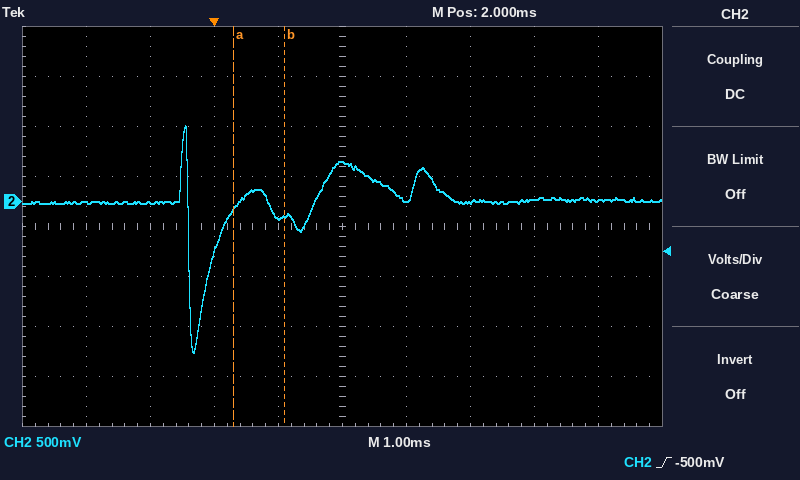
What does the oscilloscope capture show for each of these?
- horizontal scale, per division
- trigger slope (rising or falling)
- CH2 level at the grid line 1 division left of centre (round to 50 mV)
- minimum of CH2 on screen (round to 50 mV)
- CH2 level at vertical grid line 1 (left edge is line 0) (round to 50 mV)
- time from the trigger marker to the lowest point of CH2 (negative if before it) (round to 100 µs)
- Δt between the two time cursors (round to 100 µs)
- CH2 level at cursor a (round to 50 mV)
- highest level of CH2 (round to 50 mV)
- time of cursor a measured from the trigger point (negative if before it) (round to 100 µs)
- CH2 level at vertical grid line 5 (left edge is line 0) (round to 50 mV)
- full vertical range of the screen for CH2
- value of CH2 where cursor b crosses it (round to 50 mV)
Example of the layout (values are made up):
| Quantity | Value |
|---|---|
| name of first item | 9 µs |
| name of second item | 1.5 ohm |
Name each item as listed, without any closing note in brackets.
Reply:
| Quantity | Value |
|---|---|
| horizontal scale, per division | 1 ms |
| trigger slope | rising |
| CH2 level at the grid line 1 division left of centre | -150 mV |
| minimum of CH2 on screen | -1.50 V |
| CH2 level at vertical grid line 1 (left edge is line 0) | 0 mV |
| time from the trigger marker to the lowest point of CH2 (negative if before it) | -300 µs |
| Δt between the two time cursors | 800 µs |
| CH2 level at cursor a | -100 mV |
| highest level of CH2 | 750 mV |
| time of cursor a measured from the trigger point (negative if before it) | +300 µs |
| CH2 level at vertical grid line 5 (left edge is line 0) | 400 mV |
| full vertical range of the screen for CH2 | 4 V |
| value of CH2 where cursor b crosses it | -150 mV |
